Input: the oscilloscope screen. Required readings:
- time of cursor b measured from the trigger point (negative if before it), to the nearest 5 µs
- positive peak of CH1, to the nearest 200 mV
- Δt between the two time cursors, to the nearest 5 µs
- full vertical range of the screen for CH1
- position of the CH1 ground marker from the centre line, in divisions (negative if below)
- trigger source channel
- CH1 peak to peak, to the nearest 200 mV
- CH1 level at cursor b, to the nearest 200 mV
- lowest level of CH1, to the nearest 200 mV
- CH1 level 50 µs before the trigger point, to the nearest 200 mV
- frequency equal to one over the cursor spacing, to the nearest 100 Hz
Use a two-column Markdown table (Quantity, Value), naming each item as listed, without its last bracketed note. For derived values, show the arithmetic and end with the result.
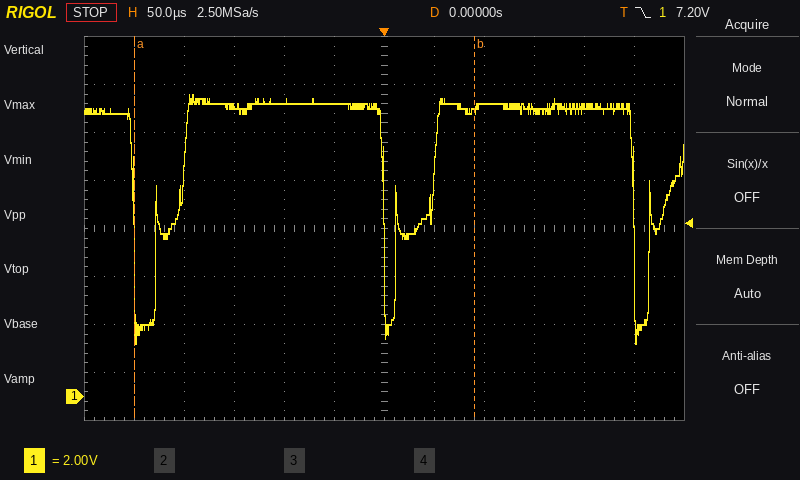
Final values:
| Quantity | Value |
|---|---|
| time of cursor b measured from the trigger point (negative if before it), to the nearest 5 µs | +90 µs |
| positive peak of CH1, to the nearest 200 mV | 12.6 V |
| Δt between the two time cursors, to the nearest 5 µs | 340 µs |
| full vertical range of the screen for CH1 | 16 V |
| position of the CH1 ground marker from the centre line, in divisions | -3.5 div |
| trigger source channel | CH1 |
| CH1 peak to peak, to the nearest 200 mV | 12.6 V − (2.2 V) = 10.4 V |
| CH1 level at cursor b, to the nearest 200 mV | 12.0 V |
| lowest level of CH1, to the nearest 200 mV | 2.2 V |
| CH1 level 50 µs before the trigger point, to the nearest 200 mV | 12.2 V |
| frequency equal to one over the cursor spacing, to the nearest 100 Hz | 1 / 340 µs ≈ 2.9 kHz |
